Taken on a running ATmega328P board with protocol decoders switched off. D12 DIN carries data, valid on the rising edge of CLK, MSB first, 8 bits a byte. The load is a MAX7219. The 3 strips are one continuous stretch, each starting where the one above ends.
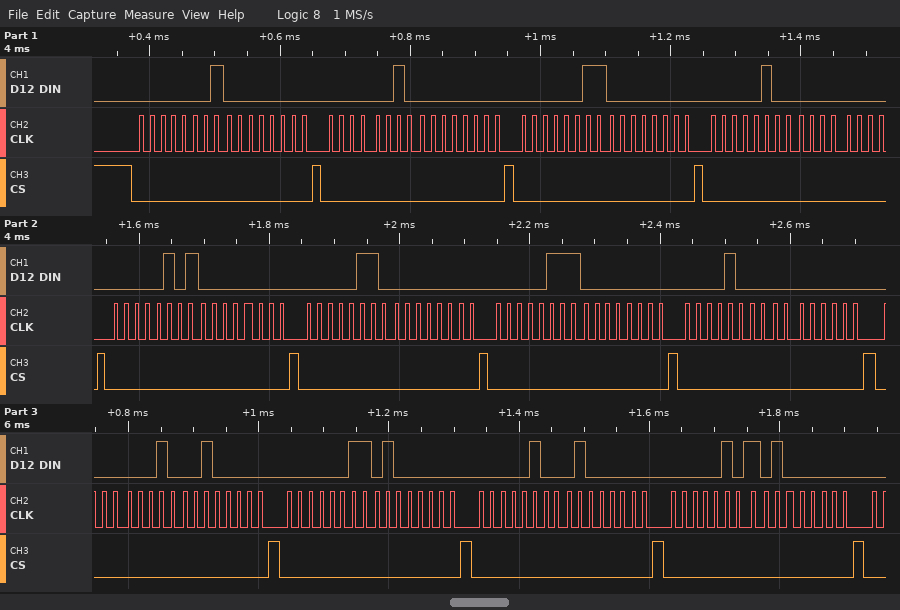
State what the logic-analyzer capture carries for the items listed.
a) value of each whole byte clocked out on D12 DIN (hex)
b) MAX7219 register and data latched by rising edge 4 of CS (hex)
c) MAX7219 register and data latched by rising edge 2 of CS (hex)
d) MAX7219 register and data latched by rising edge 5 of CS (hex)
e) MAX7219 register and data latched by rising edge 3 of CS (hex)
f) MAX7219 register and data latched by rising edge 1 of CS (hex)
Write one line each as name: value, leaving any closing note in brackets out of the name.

value of each whole byte clocked out on D12 DIN: 0x01 0x00 0x02 0x00 0x03 0x00 0x04 0x00 0x05 0x00 0x06 0x00 0x07 0x00 0x08 0x00 0x02 0x20 0x03 0x40 0x04 0x40 0x05 0x40
MAX7219 register and data latched by rising edge 4 of CS: register 0x4, data 0x00
MAX7219 register and data latched by rising edge 2 of CS: register 0x2, data 0x00
MAX7219 register and data latched by rising edge 5 of CS: register 0x5, data 0x00
MAX7219 register and data latched by rising edge 3 of CS: register 0x3, data 0x00
MAX7219 register and data latched by rising edge 1 of CS: register 0x1, data 0x00
